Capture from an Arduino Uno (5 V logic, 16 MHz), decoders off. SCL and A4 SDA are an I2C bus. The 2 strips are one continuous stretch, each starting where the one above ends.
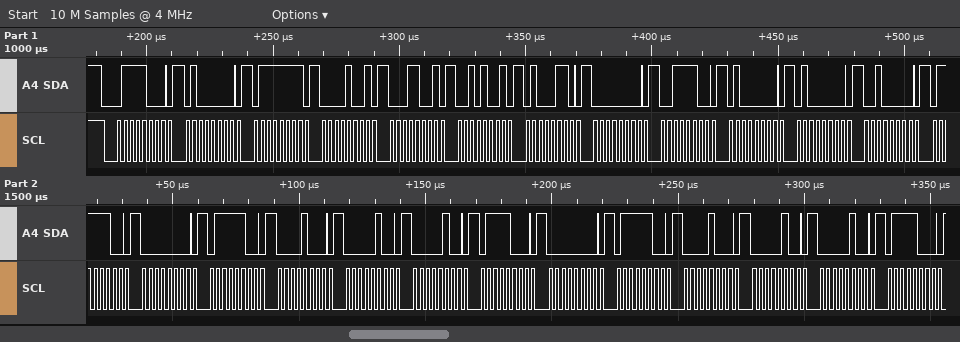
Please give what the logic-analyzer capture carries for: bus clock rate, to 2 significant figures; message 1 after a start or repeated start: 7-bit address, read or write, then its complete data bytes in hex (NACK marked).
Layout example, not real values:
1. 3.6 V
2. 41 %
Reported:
1. 400 kHz
2. 0x3C write: 40 7F 09 19 29 46 00 3C 40 40 20 7C 00 7C 08 04 04 78 00 7C 08 04 04 78
